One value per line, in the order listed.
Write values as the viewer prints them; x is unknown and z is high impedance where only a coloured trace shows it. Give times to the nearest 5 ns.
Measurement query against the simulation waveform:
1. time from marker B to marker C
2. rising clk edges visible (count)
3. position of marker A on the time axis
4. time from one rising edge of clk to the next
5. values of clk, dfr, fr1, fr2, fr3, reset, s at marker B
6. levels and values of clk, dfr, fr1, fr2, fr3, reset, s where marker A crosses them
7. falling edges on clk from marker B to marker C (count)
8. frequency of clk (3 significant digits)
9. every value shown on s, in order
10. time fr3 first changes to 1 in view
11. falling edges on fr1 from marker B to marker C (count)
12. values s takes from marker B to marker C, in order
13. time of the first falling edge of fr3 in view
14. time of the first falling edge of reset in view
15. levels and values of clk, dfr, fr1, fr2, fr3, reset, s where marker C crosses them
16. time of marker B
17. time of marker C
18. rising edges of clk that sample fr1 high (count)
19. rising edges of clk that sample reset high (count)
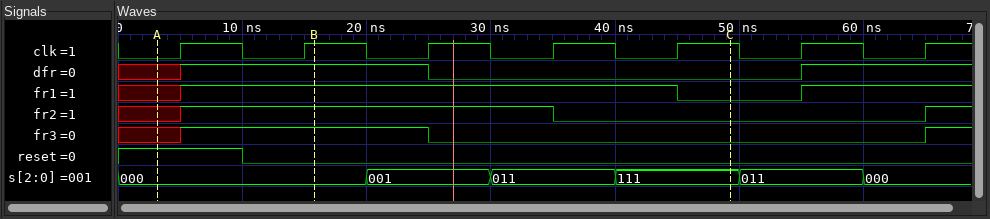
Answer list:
35 ns
7
5 ns
10 ns
clk=1, dfr=1, fr1=1, fr2=1, fr3=1, reset=0, s=000
clk=0, dfr=x, fr1=x, fr2=x, fr3=x, reset=1, s=000
3
100 MHz
000, 001, 011, 111, 011, 000
5 ns
1
000, 001, 011, 111
25 ns
10 ns
clk=1, dfr=0, fr1=0, fr2=0, fr3=0, reset=0, s=111
15 ns
50 ns
5
1
